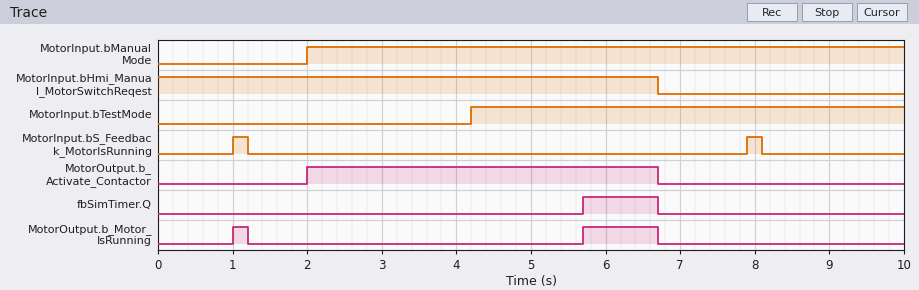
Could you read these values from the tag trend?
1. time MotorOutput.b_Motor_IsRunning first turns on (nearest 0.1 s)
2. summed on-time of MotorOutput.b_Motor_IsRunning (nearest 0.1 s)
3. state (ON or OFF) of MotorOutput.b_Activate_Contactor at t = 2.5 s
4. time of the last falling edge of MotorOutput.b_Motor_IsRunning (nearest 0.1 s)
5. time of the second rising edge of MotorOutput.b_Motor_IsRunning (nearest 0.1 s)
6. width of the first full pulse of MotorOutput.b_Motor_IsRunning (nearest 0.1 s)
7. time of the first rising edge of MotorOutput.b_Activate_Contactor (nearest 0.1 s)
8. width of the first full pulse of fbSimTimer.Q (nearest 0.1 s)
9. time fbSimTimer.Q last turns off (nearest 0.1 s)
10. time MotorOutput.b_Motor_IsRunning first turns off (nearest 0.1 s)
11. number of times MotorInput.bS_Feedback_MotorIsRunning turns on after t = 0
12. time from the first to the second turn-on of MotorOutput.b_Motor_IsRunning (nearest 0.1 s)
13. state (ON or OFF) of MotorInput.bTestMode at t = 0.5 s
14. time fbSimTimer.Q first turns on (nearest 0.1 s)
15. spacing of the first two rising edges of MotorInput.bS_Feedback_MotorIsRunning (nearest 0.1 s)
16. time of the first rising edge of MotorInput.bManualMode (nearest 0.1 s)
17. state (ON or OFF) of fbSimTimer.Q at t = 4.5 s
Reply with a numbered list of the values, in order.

1. 1.0 s
2. 1.2 s
3. ON
4. 6.7 s
5. 5.7 s
6. 0.2 s
7. 2.0 s
8. 1.0 s
9. 6.7 s
10. 1.2 s
11. 2
12. 4.7 s
13. OFF
14. 5.7 s
15. 6.9 s
16. 2.0 s
17. OFF
